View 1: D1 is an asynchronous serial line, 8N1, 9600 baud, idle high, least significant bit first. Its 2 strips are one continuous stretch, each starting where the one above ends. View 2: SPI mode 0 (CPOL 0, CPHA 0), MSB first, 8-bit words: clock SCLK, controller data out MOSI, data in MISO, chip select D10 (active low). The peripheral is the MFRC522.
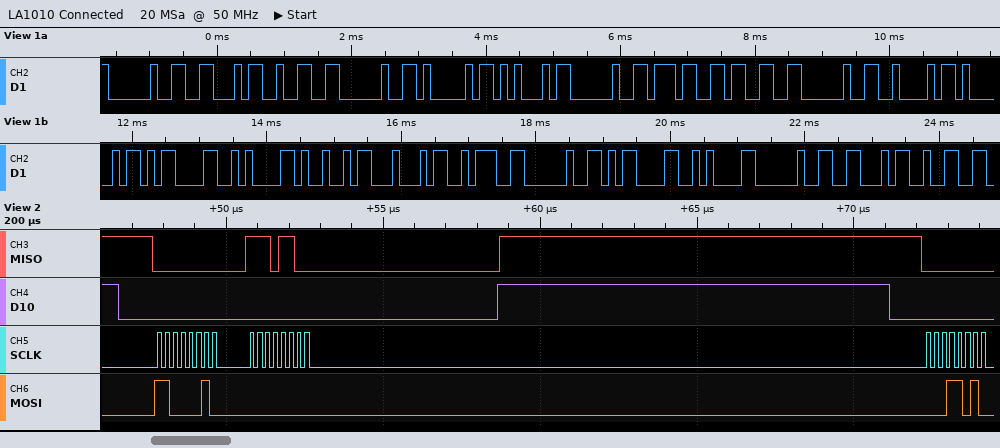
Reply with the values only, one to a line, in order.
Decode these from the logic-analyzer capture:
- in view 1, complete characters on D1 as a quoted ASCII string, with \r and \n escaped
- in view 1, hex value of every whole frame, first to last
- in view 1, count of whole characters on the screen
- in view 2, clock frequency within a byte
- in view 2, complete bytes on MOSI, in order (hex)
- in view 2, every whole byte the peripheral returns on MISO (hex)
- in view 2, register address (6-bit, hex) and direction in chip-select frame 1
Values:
" F2 AE 73 BA\r\nID: \r\n F2"
20 46 32 20 41 45 20 37 33 20 42 41 0D 0A 49 44 3A 20 0D 0A 20 46 32
23
4 MHz
C2 00 1A
00 EC 00
0x21 read
